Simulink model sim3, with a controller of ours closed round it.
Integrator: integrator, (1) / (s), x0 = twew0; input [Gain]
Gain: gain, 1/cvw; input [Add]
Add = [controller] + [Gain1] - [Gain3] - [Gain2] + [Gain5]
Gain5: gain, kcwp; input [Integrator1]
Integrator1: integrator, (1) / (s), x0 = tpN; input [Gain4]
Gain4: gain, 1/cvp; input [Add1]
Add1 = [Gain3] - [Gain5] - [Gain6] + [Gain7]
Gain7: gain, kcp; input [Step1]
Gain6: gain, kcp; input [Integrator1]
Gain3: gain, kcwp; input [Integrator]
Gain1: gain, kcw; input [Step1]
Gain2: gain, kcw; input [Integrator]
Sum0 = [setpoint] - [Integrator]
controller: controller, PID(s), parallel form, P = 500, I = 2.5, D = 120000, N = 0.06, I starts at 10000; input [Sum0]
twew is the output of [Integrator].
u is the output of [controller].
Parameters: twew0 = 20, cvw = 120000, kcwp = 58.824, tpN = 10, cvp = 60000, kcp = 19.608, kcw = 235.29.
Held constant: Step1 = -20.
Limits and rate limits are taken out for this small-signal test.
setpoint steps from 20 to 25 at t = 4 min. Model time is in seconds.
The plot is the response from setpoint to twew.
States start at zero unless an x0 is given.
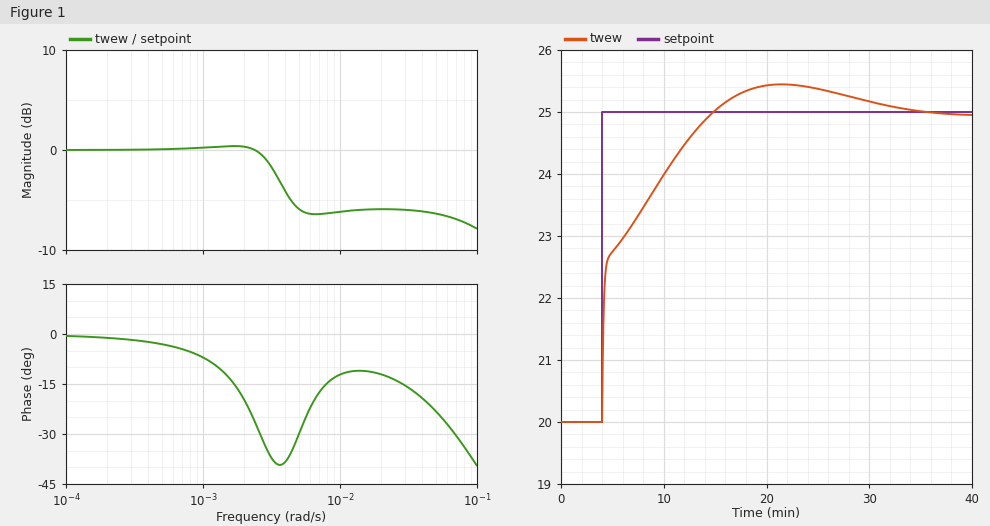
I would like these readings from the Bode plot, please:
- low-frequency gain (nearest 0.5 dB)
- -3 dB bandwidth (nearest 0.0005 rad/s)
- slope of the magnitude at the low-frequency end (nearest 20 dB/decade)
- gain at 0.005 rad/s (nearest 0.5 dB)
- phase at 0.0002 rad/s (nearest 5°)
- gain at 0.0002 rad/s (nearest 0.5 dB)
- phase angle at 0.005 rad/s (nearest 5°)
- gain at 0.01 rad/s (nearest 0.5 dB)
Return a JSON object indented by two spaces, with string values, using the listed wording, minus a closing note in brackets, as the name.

{
  "low-frequency gain": "0.0 dB",
  "-3 dB bandwidth": "0.0035 rad/s",
  "slope of the magnitude at the low-frequency end": "0 dB/decade",
  "gain at 0.005 rad/s": "-6.0 dB",
  "phase at 0.0002 rad/s": "0°",
  "gain at 0.0002 rad/s": "0.0 dB",
  "phase angle at 0.005 rad/s": "-30°",
  "gain at 0.01 rad/s": "-6.0 dB"
}
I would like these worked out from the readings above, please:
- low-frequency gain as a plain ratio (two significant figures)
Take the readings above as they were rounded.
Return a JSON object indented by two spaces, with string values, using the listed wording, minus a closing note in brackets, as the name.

{
  "low-frequency gain as a plain ratio": "1.0"
}
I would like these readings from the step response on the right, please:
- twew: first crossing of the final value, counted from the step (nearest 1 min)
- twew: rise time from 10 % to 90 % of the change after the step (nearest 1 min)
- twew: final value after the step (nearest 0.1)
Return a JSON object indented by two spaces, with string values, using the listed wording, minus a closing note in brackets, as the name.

{
  "twew: first crossing of the final value, counted from the step": "11 min",
  "twew: rise time from 10 % to 90 % of the change after the step": "8 min",
  "twew: final value after the step": "25.0"
}
